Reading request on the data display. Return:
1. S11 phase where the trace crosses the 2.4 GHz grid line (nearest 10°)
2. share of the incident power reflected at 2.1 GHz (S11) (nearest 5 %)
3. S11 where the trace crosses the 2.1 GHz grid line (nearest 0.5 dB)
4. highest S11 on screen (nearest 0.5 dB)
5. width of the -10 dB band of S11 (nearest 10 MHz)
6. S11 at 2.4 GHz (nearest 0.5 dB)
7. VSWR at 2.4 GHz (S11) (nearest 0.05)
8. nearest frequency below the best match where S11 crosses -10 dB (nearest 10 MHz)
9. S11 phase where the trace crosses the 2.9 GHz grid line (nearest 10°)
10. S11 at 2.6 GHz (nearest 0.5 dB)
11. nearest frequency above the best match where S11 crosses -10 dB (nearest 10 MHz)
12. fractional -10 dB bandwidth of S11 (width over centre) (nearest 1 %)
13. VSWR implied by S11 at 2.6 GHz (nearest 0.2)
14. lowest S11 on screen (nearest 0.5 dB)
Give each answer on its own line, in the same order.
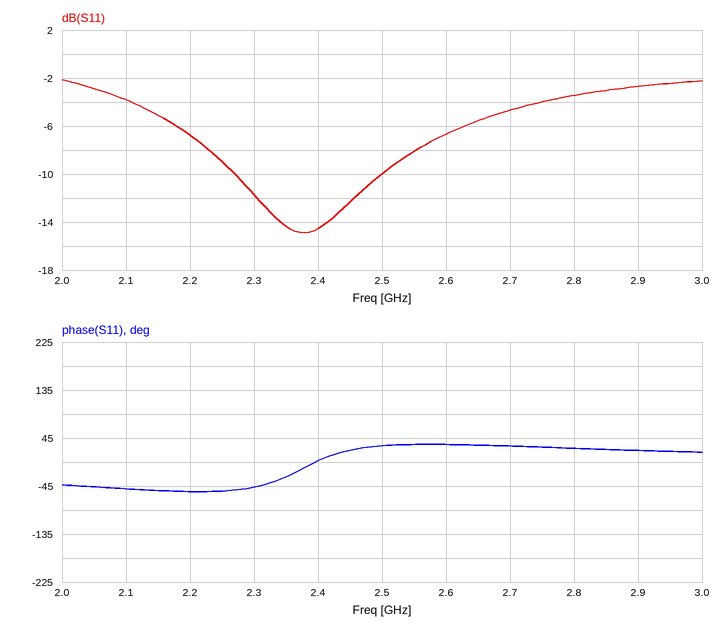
0°
40 %
-4.0 dB
-2.0 dB
230 MHz
-14.5 dB
1.45
2.27 GHz
20°
-6.5 dB
2.50 GHz
10 %
2.8
-15.0 dB
